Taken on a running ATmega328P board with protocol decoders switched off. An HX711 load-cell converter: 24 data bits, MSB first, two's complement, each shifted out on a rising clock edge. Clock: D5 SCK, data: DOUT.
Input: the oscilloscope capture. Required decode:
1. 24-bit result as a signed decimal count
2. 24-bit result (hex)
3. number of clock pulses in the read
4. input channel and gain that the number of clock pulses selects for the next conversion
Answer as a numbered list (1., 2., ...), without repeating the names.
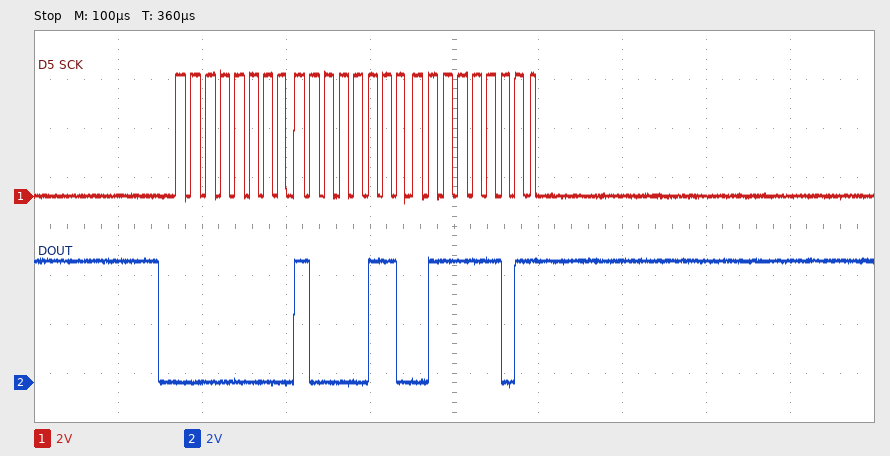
1. 34429
2. 0x00867D
3. 25
4. channel A, gain 128
